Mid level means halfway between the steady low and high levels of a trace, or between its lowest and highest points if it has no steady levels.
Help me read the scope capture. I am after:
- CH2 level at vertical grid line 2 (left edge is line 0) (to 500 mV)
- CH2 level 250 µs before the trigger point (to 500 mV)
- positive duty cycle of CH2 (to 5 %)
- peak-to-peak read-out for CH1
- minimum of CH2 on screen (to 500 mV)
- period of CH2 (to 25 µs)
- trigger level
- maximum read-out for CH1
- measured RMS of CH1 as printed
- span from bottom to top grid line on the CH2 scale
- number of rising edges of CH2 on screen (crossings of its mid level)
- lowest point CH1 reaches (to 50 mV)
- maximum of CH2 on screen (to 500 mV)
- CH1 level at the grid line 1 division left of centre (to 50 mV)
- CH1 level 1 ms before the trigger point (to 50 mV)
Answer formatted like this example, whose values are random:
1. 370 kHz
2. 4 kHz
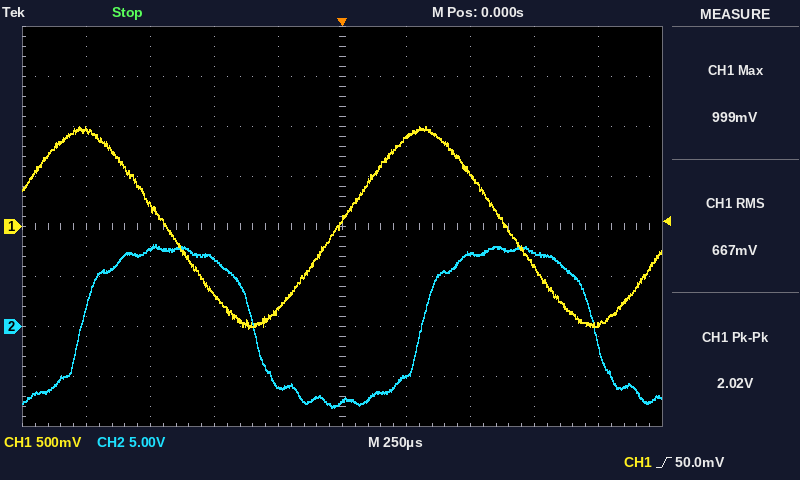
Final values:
1. 8.0 V
2. -6.0 V
3. 50 %
4. 2.02 V
5. -8.0 V
6. 1.325 ms
7. 50.0 mV
8. 999 mV
9. 667 mV
10. 40 V
11. 2
12. -1.00 V
13. 8.0 V
14. -850 mV
15. 950 mV
